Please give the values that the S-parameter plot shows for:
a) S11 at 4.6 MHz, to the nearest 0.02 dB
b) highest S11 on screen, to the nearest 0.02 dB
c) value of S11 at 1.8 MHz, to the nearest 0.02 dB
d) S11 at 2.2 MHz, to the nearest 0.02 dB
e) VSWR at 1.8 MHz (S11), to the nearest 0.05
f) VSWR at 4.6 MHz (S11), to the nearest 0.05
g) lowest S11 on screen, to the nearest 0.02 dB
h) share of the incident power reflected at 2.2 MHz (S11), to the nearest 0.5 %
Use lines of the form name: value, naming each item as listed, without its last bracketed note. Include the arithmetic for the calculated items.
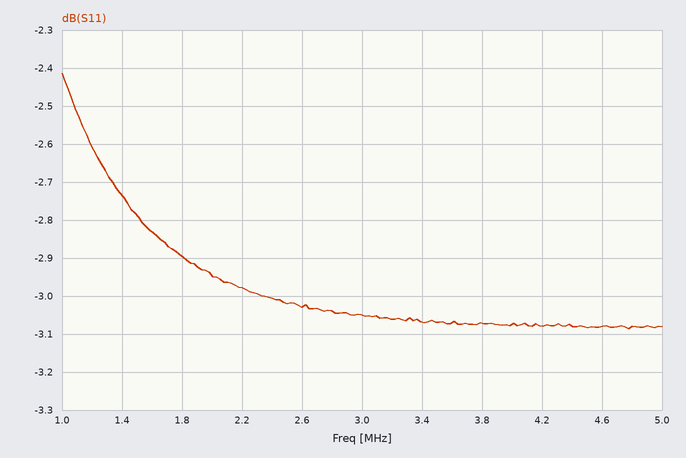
S11 at 4.6 MHz, to the nearest 0.02 dB: -3.08 dB
highest S11 on screen, to the nearest 0.02 dB: -2.42 dB
value of S11 at 1.8 MHz, to the nearest 0.02 dB: -2.90 dB
S11 at 2.2 MHz, to the nearest 0.02 dB: -2.98 dB
VSWR at 1.8 MHz (S11), to the nearest 0.05: |Γ| = 10^(-2.9/20) = 0.7161; VSWR = (1 + 0.7161)/(1 − 0.7161) ≈ 6.05
VSWR at 4.6 MHz (S11), to the nearest 0.05: |Γ| = 10^(-3.08/20) = 0.7015; VSWR = (1 + 0.7015)/(1 − 0.7015) ≈ 5.70
lowest S11 on screen, to the nearest 0.02 dB: -3.08 dB
share of the incident power reflected at 2.2 MHz (S11), to the nearest 0.5 %: 10^(-2.98/10) ≈ 50.4 %, so 50.5 % to the nearest 0.5 %
